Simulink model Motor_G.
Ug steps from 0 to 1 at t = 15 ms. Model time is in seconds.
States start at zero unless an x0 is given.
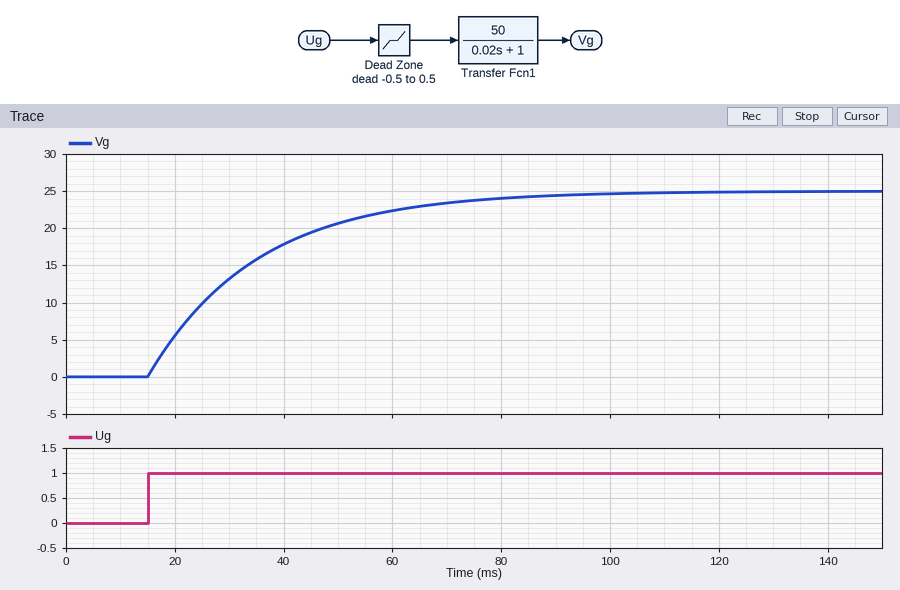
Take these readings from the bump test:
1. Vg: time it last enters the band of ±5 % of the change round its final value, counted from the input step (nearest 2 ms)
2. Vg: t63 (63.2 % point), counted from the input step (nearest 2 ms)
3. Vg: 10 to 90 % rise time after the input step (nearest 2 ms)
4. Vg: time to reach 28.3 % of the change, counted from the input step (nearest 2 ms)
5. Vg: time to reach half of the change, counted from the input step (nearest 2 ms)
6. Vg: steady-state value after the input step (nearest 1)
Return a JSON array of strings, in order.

["60 ms", "20 ms", "44 ms", "6 ms", "14 ms", "25"]
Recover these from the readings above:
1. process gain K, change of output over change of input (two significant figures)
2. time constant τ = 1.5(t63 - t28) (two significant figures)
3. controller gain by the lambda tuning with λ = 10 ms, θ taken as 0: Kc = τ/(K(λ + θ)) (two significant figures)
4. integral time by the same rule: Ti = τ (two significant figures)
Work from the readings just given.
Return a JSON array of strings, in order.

["25", "21 ms", "0.084", "21 ms"]
